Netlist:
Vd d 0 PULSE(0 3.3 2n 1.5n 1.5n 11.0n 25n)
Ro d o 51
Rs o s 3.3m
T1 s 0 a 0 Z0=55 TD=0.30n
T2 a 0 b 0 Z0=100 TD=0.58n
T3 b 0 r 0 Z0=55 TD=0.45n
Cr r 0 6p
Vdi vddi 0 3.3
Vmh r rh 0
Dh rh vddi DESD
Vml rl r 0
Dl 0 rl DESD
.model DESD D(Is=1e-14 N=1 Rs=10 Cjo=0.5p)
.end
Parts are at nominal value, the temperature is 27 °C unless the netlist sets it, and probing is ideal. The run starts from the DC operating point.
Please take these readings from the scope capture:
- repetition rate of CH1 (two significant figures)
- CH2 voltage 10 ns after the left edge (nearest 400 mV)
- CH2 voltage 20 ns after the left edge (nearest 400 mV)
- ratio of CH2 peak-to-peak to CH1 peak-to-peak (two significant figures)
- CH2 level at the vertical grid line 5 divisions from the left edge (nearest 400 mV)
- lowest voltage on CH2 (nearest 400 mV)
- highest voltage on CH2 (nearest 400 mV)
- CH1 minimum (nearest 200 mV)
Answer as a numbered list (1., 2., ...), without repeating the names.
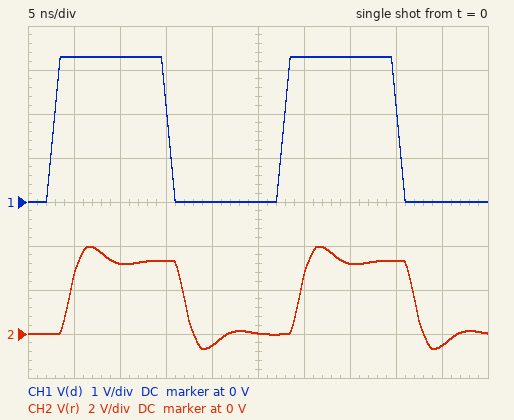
1. 40 MHz
2. 3.2 V
3. -400 mV
4. 1.4
5. 0 V
6. -800 mV
7. 4.0 V
8. 0 V
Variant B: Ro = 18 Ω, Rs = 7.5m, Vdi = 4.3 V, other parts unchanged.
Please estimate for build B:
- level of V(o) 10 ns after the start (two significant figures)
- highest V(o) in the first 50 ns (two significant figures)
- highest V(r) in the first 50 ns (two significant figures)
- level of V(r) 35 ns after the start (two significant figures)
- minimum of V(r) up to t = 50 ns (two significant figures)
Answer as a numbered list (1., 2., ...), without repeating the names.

1. 3.5 V
2. 3.7 V
3. 5.2 V
4. 2.4 V
5. -1.0 V
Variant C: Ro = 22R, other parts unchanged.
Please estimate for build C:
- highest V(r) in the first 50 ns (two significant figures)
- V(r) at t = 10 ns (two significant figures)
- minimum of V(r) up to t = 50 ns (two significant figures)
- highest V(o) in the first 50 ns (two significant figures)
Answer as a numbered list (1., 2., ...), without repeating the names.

1. 4.3 V
2. 3.2 V
3. -980 mV
4. 3.5 V
